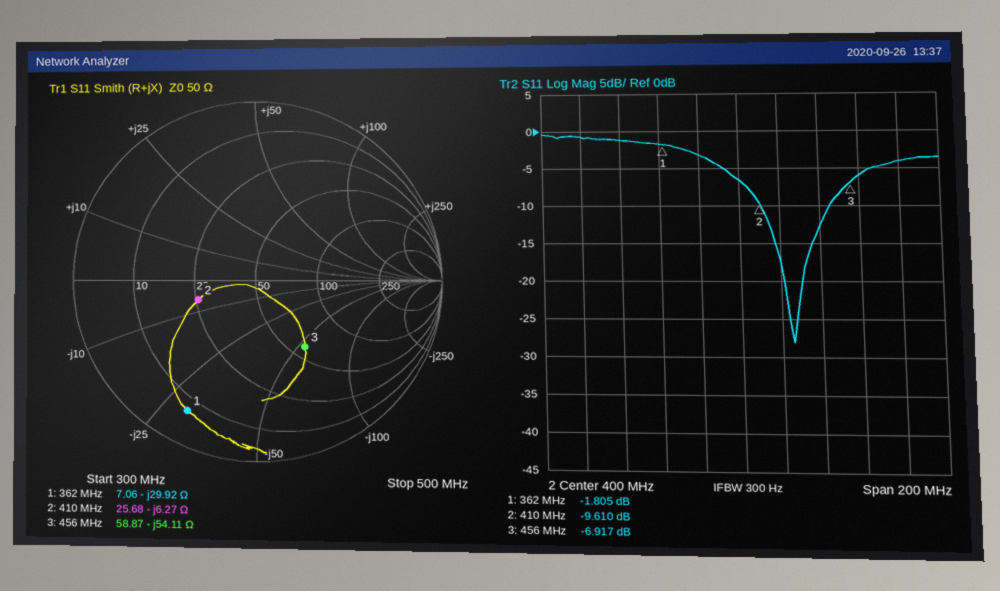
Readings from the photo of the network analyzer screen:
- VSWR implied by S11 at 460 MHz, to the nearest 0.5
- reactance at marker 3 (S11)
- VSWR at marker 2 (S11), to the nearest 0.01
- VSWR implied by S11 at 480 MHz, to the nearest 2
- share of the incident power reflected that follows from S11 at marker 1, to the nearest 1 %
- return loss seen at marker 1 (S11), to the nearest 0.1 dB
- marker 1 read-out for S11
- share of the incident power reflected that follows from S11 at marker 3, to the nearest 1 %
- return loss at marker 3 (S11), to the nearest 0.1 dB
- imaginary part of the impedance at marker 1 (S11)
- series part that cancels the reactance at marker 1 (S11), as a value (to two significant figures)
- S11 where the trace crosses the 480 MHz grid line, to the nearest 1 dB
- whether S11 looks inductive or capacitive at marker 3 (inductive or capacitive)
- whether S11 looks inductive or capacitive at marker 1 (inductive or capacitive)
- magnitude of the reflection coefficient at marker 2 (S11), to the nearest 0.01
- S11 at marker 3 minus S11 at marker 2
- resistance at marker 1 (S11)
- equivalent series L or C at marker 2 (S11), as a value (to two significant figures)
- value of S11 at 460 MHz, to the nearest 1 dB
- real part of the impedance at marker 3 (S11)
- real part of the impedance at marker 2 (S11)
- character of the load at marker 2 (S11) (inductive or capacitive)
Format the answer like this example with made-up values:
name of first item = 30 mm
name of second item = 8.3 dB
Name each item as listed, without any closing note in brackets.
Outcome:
VSWR implied by S11 at 460 MHz, to the nearest 0.5 = 3.0
reactance at marker 3 = -54.11 Ω
VSWR at marker 2 (S11), to the nearest 0.01 = 1.99
VSWR implied by S11 at 480 MHz, to the nearest 2 = 4
share of the incident power reflected that follows from S11 at marker 1, to the nearest 1 % = 66 %
return loss seen at marker 1 (S11), to the nearest 0.1 dB = 1.8 dB
marker 1 read-out for S11 = -1.805 dB
share of the incident power reflected that follows from S11 at marker 3, to the nearest 1 % = 20 %
return loss at marker 3 (S11), to the nearest 0.1 dB = 6.9 dB
imaginary part of the impedance at marker 1 = -29.92 Ω
series part that cancels the reactance at marker 1 (S11), as a value = 13 nH
S11 where the trace crosses the 480 MHz grid line, to the nearest 1 dB = -4 dB
whether S11 looks inductive or capacitive at marker 3 = capacitive
whether S11 looks inductive or capacitive at marker 1 = capacitive
magnitude of the reflection coefficient at marker 2 (S11), to the nearest 0.01 = 0.33
S11 at marker 3 minus S11 at marker 2 = 2.693 dB
resistance at marker 1 = 7.06 Ω
equivalent series L or C at marker 2 (S11), as a value = 62 pF
value of S11 at 460 MHz, to the nearest 1 dB = -6 dB
real part of the impedance at marker 3 = 58.87 Ω
real part of the impedance at marker 2 = 25.68 Ω
character of the load at marker 2 (S11) = capacitive
